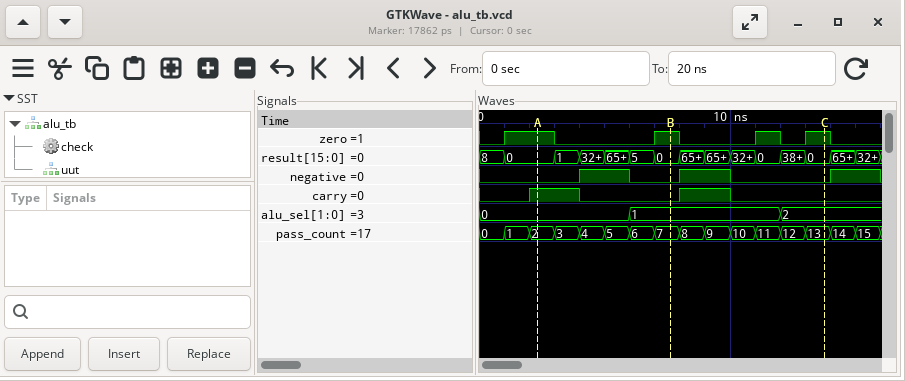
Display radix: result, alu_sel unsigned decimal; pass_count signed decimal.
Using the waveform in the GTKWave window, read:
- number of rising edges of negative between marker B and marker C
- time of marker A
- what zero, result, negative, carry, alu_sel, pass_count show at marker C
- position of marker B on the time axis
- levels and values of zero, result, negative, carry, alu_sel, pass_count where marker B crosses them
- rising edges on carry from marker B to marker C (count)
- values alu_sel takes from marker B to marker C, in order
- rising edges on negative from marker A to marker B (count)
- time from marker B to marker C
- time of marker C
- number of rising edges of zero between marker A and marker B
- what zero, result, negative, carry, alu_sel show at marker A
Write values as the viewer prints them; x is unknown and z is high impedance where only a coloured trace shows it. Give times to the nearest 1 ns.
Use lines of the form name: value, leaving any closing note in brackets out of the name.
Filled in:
number of rising edges of negative between marker B and marker C: 1
time of marker A: 2 ns
what zero, result, negative, carry, alu_sel, pass_count show at marker C: zero=1, result=0, negative=0, carry=0, alu_sel=2, pass_count=13
position of marker B on the time axis: 8 ns
levels and values of zero, result, negative, carry, alu_sel, pass_count where marker B crosses them: zero=1, result=0, negative=0, carry=0, alu_sel=1, pass_count=7
rising edges on carry from marker B to marker C: 1
values alu_sel takes from marker B to marker C, in order: 1, 2
rising edges on negative from marker A to marker B: 1
time from marker B to marker C: 6 ns
time of marker C: 14 ns
number of rising edges of zero between marker A and marker B: 1
what zero, result, negative, carry, alu_sel show at marker A: zero=1, result=0, negative=0, carry=1, alu_sel=0
